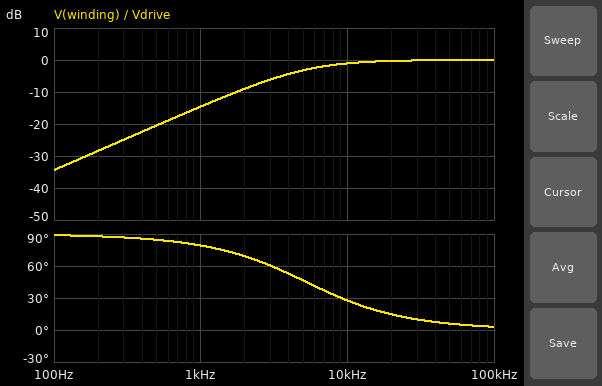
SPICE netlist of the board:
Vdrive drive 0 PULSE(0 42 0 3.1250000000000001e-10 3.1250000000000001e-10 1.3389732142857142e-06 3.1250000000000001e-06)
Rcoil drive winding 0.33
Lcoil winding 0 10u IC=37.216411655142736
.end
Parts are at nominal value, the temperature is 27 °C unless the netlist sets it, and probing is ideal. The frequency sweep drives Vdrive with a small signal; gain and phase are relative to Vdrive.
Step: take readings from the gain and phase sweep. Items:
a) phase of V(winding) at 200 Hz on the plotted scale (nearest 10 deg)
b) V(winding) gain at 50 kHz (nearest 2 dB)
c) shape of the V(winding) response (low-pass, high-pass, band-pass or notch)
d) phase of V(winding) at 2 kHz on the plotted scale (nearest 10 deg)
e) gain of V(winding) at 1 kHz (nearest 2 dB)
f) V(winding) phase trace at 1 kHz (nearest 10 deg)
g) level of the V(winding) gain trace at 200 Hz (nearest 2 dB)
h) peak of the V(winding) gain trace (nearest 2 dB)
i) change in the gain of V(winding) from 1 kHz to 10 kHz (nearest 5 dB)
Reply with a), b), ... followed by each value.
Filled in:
a) 90 deg
b) 0 dB
c) high-pass
d) 70 deg
e) -14 dB
f) 80 deg
g) -28 dB
h) 0 dB
i) 15 dB
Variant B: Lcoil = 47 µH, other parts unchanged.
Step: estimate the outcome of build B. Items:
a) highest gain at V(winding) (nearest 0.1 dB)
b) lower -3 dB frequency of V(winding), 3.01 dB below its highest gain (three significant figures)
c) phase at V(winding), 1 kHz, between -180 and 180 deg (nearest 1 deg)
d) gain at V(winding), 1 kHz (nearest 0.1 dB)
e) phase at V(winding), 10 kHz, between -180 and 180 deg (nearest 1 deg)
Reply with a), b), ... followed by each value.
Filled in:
a) 0 dB
b) 1.12 kHz
c) 48 deg
d) -3.5 dB
e) 6 deg
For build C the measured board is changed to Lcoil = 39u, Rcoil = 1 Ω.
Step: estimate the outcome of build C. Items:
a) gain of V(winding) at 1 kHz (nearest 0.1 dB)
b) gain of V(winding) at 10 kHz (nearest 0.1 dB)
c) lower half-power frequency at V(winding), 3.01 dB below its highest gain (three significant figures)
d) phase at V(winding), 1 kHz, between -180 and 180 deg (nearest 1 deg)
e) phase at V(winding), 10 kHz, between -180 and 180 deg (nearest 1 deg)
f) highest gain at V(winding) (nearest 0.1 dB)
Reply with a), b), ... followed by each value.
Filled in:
a) -12.5 dB
b) -0.7 dB
c) 4.08 kHz
d) 76 deg
e) 22 deg
f) 0 dB
